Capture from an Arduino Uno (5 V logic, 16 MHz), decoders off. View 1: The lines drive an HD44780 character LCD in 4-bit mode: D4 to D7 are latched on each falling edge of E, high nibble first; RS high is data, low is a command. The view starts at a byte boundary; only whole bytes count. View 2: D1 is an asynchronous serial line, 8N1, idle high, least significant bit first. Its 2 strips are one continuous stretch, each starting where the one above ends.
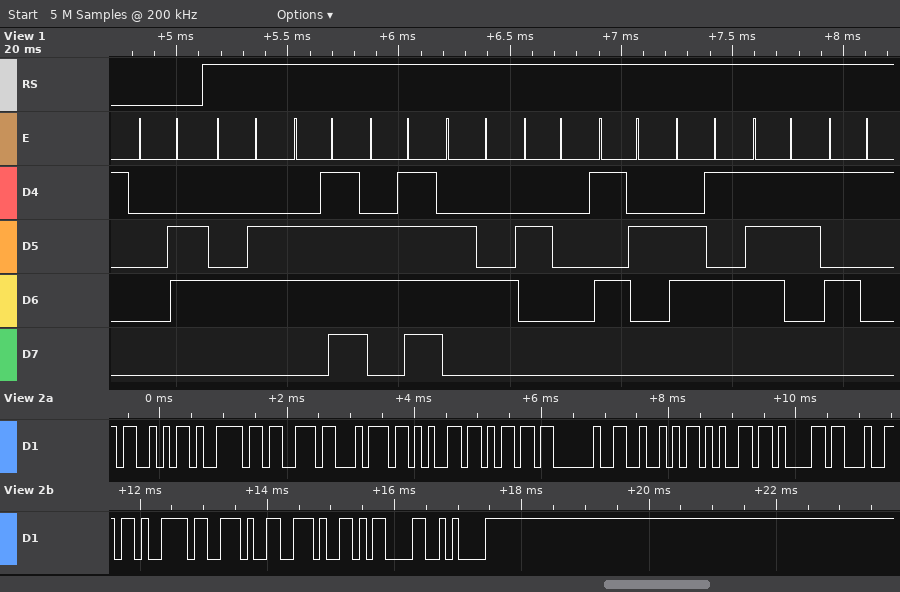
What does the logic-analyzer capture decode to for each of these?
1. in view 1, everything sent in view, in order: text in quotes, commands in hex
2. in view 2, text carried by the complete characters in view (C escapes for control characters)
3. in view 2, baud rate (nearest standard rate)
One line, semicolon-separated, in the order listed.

0x06 "Food ResQ"; "System Ready..\r\n"; 9600 baud
